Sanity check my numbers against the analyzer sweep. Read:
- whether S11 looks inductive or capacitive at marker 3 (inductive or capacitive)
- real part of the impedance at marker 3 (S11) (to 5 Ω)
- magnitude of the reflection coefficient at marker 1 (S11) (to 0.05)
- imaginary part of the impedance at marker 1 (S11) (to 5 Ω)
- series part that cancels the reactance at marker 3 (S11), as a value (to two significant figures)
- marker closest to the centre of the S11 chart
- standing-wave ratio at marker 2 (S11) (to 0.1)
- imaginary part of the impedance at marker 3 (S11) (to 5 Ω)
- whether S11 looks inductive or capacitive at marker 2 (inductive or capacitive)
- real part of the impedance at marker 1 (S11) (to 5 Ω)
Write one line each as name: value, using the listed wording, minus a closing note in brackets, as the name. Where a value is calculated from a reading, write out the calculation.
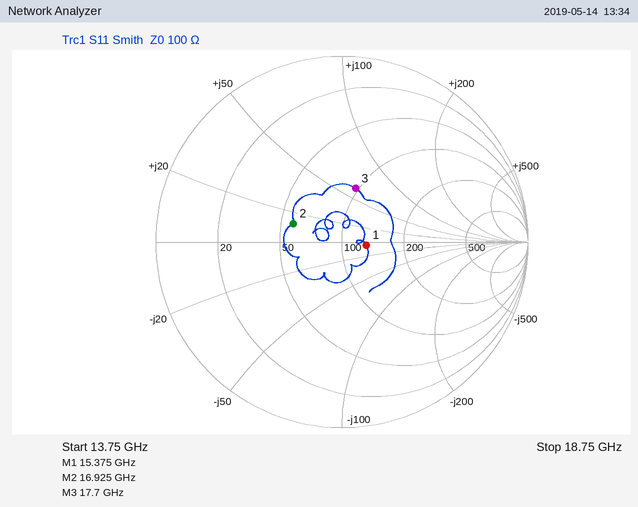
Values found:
whether S11 looks inductive or capacitive at marker 3: inductive
real part of the impedance at marker 3 (S11): 95 Ω
magnitude of the reflection coefficient at marker 1 (S11): 0.15
imaginary part of the impedance at marker 1 (S11): -5 Ω
series part that cancels the reactance at marker 3 (S11), as a value: C = 1/(2π × 17.7 GHz × 60 Ω) ≈ 150 fF
marker closest to the centre of the S11 chart: marker 1
standing-wave ratio at marker 2 (S11): 1.8
imaginary part of the impedance at marker 3 (S11): +60 Ω
whether S11 looks inductive or capacitive at marker 2: inductive
real part of the impedance at marker 1 (S11): 130 Ω
